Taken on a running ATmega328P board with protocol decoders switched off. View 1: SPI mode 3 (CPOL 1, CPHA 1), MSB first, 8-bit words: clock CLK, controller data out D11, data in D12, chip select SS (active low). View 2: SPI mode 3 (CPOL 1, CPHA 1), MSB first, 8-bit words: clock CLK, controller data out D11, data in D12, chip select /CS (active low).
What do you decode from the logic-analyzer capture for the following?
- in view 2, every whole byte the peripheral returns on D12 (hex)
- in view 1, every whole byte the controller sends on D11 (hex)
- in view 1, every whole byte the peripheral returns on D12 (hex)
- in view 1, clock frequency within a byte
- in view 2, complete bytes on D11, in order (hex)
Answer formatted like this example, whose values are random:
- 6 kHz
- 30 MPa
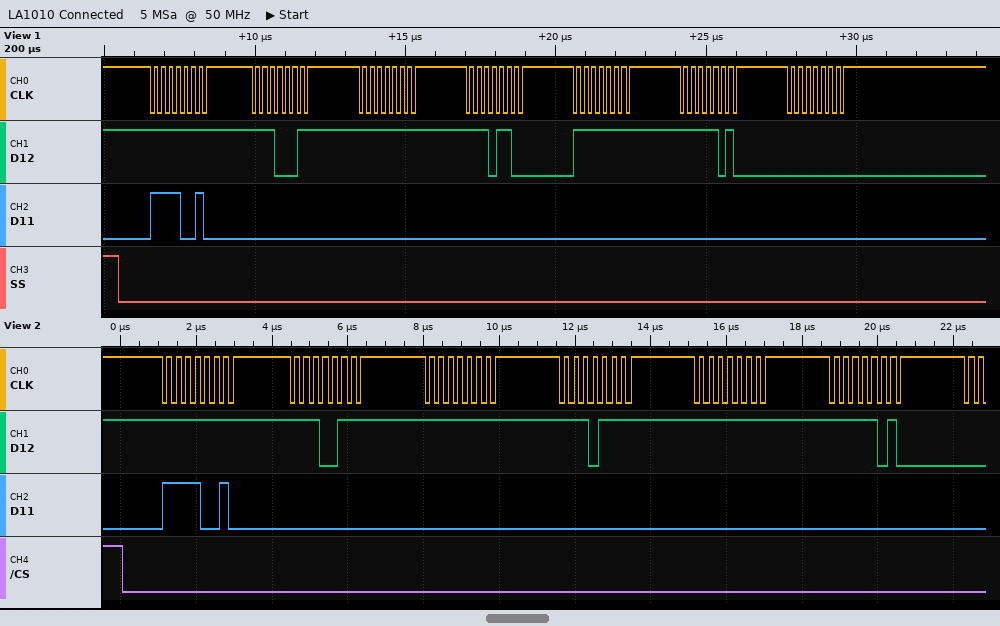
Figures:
- FF E7 FF EF FF FA
- F2 00 00 00 00 00 00
- FF E3 FF EC FF FA 00
- 4 MHz
- F2 00 00 00 00 00
